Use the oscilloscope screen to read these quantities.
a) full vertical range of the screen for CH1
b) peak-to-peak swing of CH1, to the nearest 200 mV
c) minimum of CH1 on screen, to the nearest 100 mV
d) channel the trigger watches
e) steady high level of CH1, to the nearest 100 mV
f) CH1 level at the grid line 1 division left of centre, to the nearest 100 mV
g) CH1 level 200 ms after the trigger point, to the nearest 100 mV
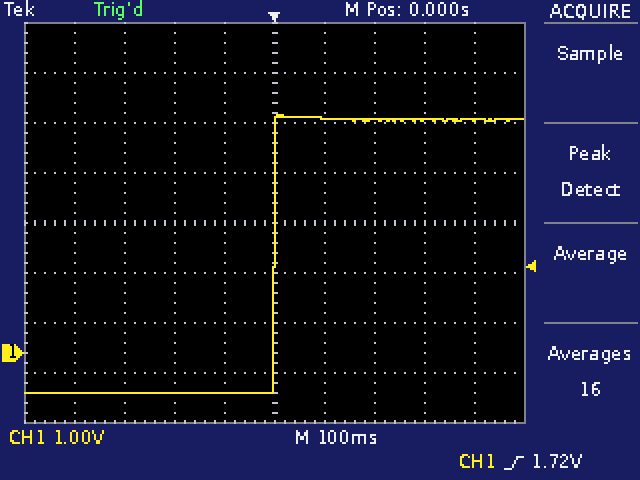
8 V
5.6 V
-800 mV
CH1
4.7 V
-800 mV
4.7 V
